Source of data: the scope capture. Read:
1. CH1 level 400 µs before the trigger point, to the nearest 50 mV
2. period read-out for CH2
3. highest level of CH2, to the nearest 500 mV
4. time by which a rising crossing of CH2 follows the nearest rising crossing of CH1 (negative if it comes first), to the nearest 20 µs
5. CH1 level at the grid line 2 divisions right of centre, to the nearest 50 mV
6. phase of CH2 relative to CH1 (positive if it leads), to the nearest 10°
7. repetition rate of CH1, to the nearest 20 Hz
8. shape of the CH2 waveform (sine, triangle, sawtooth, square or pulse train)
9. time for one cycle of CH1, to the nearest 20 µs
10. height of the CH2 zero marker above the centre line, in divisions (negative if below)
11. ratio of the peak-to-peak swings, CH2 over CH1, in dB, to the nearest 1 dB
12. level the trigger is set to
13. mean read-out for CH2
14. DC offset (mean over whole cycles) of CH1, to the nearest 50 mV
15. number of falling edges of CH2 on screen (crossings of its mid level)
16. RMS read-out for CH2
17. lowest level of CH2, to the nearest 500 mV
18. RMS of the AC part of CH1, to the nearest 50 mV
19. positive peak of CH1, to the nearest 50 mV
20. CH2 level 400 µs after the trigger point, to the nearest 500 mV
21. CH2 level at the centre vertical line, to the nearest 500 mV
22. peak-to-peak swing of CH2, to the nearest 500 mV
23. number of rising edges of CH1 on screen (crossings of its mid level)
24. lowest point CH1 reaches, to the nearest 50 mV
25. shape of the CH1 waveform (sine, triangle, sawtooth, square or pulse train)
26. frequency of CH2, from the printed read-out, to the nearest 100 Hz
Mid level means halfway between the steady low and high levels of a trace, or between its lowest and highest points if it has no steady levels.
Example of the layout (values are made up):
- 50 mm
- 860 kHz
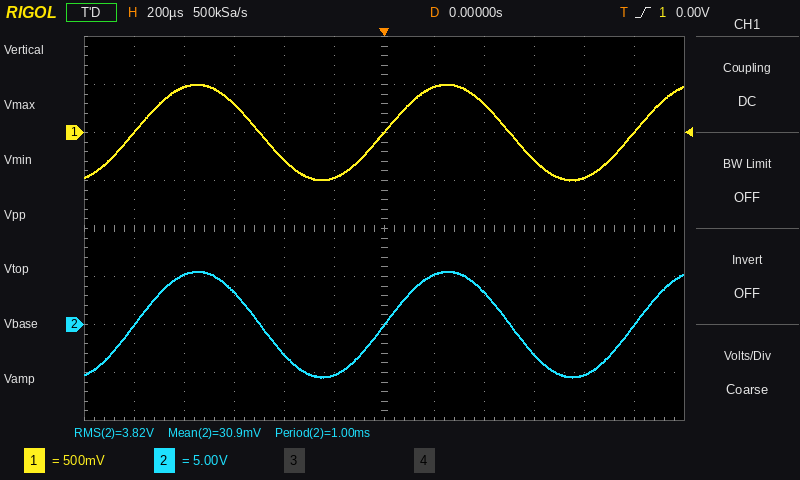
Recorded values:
- -300 mV
- 1.00 ms
- 5.5 V
- 0 µs
- 300 mV
- 0°
- 1.00 kHz
- sine
- 1.00 ms
- -2.0 div
- 21 dB
- 0.00 V
- 30.9 mV
- 0 mV
- 2
- 3.82 V
- -5.5 V
- 350 mV
- 500 mV
- 3.5 V
- 0.0 V
- 11.0 V
- 3
- -500 mV
- sine
- 1.0 kHz
